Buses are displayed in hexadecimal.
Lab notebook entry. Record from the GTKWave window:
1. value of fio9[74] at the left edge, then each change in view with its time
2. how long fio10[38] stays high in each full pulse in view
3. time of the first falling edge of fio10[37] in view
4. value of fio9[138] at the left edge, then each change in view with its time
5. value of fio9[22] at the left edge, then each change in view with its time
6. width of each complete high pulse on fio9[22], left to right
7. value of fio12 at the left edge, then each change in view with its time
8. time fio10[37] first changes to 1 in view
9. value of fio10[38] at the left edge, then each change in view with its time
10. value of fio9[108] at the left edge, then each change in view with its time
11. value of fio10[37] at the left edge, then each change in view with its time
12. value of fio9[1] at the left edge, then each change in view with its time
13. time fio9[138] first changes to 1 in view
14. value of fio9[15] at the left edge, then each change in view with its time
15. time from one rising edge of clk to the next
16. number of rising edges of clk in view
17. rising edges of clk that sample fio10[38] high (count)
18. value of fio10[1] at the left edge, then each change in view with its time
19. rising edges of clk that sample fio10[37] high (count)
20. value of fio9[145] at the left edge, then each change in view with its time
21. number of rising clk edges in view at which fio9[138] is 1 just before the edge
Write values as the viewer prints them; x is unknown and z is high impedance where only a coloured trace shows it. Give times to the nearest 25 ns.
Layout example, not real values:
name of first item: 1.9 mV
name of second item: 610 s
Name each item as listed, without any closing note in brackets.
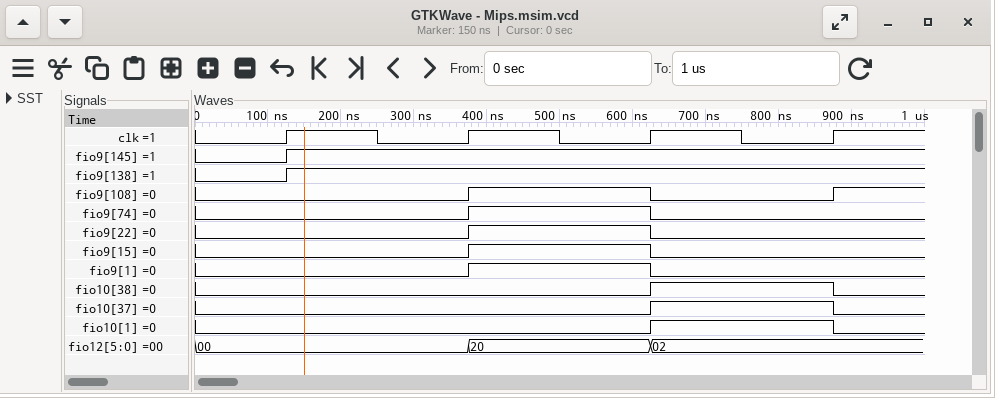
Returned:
value of fio9[74] at the left edge, then each change in view with its time: 0, 1 at 375 ns, 0 at 625 ns
how long fio10[38] stays high in each full pulse in view: 250 ns
time of the first falling edge of fio10[37] in view: 875 ns
value of fio9[138] at the left edge, then each change in view with its time: 0, 1 at 125 ns
value of fio9[22] at the left edge, then each change in view with its time: 0, 1 at 375 ns, 0 at 625 ns
width of each complete high pulse on fio9[22], left to right: 250 ns
value of fio12 at the left edge, then each change in view with its time: 00, 20 at 375 ns, 02 at 625 ns
time fio10[37] first changes to 1 in view: 625 ns
value of fio10[38] at the left edge, then each change in view with its time: 0, 1 at 625 ns, 0 at 875 ns
value of fio9[108] at the left edge, then each change in view with its time: 0, 1 at 375 ns, 0 at 625 ns, 1 at 875 ns
value of fio10[37] at the left edge, then each change in view with its time: 0, 1 at 625 ns, 0 at 875 ns
value of fio9[1] at the left edge, then each change in view with its time: 0, 1 at 375 ns, 0 at 625 ns
time fio9[138] first changes to 1 in view: 125 ns
value of fio9[15] at the left edge, then each change in view with its time: 0, 1 at 375 ns, 0 at 625 ns
time from one rising edge of clk to the next: 250 ns
number of rising edges of clk in view: 4
rising edges of clk that sample fio10[38] high: 1
value of fio10[1] at the left edge, then each change in view with its time: 0, 1 at 625 ns, 0 at 875 ns
rising edges of clk that sample fio10[37] high: 1
value of fio9[145] at the left edge, then each change in view with its time: 0, 1 at 125 ns
number of rising clk edges in view at which fio9[138] is 1 just before the edge: 3
